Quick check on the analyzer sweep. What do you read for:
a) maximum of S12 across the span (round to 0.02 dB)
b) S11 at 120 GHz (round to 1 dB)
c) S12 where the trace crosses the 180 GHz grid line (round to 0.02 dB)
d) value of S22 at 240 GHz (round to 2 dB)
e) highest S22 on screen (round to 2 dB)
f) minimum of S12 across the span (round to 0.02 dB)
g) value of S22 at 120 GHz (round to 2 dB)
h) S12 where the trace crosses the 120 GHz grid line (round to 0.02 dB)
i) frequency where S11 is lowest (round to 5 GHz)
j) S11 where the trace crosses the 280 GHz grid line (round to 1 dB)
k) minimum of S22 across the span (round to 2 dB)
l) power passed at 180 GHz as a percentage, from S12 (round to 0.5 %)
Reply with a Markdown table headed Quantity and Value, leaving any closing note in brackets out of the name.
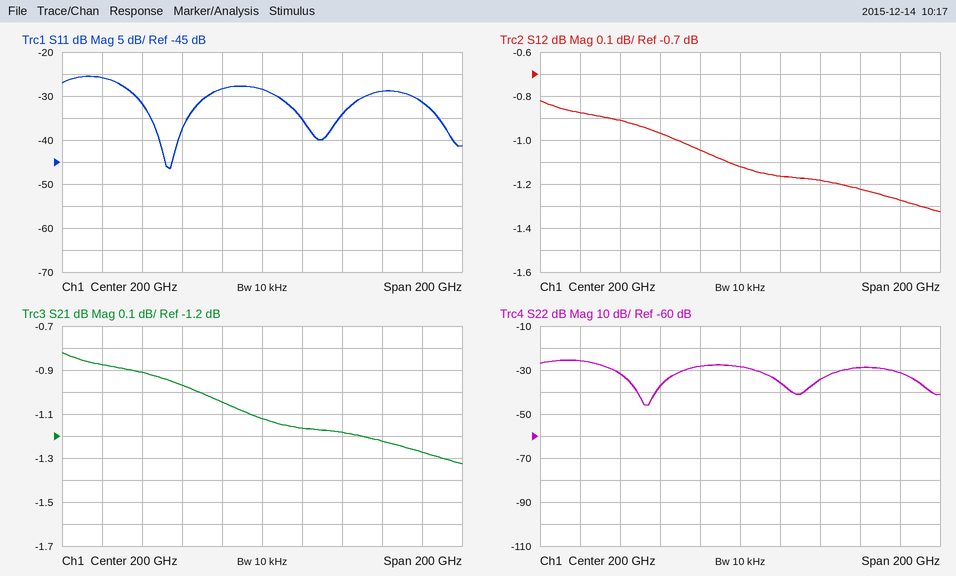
| Quantity | Value |
|---|---|
| maximum of S12 across the span | -0.82 dB |
| S11 at 120 GHz | -26 dB |
| S12 where the trace crosses the 180 GHz grid line | -1.04 dB |
| value of S22 at 240 GHz | -34 dB |
| highest S22 on screen | -26 dB |
| minimum of S12 across the span | -1.32 dB |
| value of S22 at 120 GHz | -26 dB |
| S12 where the trace crosses the 120 GHz grid line | -0.88 dB |
| frequency where S11 is lowest | 155 GHz |
| S11 where the trace crosses the 280 GHz grid line | -31 dB |
| minimum of S22 across the span | -46 dB |
| power passed at 180 GHz as a percentage, from S12 | 78.5 % |
